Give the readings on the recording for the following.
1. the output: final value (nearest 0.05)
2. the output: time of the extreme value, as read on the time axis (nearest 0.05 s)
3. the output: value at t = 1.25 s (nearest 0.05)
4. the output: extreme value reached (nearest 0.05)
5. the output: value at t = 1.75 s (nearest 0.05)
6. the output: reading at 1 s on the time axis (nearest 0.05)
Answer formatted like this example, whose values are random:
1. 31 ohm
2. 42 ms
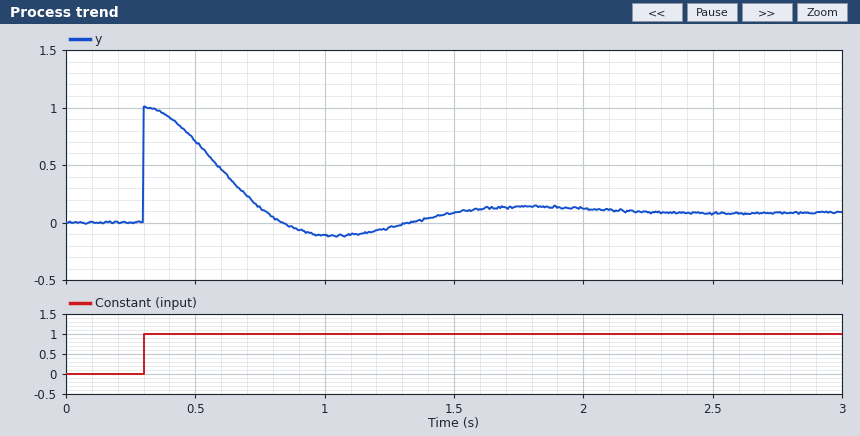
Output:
1. 0.10
2. 0.30 s
3. -0.05
4. 1.00
5. 0.15
6. -0.10
